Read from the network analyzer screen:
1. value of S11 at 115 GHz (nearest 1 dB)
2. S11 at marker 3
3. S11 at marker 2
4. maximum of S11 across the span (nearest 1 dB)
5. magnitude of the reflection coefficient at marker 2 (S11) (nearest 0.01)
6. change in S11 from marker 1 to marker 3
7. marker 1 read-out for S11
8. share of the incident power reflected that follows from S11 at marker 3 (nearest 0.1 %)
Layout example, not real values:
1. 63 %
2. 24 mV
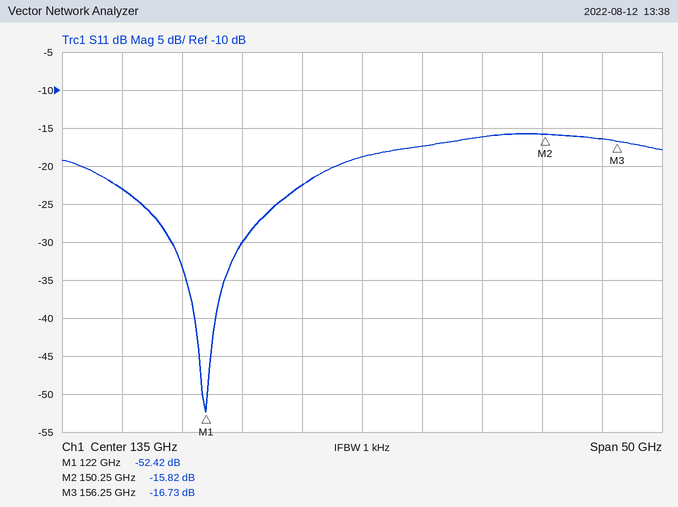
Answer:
1. -23 dB
2. -16.73 dB
3. -15.82 dB
4. -16 dB
5. 0.16
6. 35.69 dB
7. -52.42 dB
8. 2.1 %
